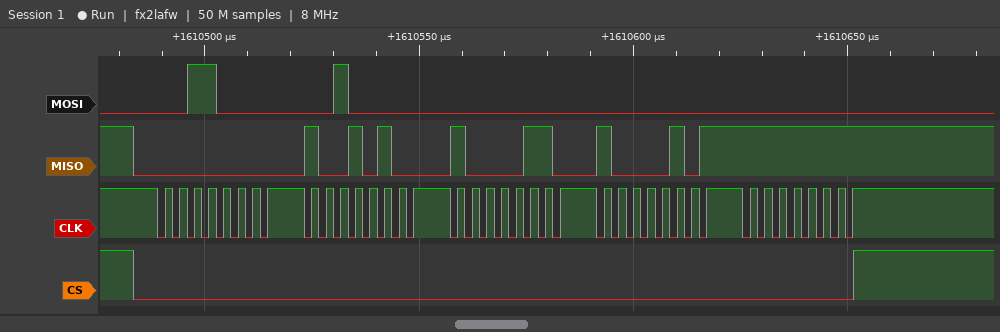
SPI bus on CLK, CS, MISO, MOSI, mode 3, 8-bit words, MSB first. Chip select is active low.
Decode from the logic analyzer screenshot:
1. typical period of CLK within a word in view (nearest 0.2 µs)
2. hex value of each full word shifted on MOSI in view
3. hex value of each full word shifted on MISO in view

3.4 µs
30, 20, 00, 00, 00
00, 94, 86, 85, FF
